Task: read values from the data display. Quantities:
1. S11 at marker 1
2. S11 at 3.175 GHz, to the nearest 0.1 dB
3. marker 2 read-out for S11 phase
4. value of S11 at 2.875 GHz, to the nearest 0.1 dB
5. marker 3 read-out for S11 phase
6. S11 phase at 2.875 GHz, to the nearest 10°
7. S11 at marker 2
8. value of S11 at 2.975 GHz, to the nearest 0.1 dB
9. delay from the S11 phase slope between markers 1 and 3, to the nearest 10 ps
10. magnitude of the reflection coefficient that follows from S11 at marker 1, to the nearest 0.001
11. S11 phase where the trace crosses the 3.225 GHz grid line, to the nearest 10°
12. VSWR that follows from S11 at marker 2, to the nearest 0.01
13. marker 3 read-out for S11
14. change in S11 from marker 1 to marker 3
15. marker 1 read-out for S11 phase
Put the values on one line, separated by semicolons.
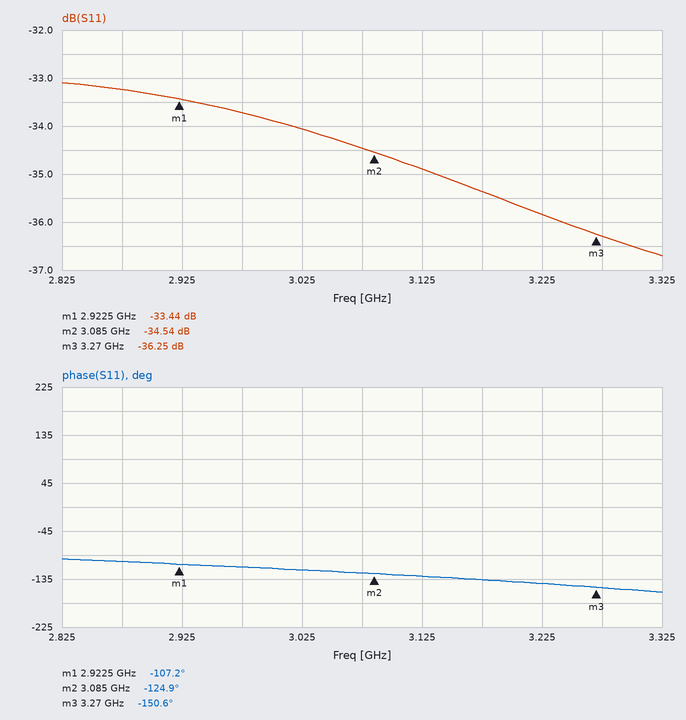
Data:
-33.44 dB; -35.4 dB; -124.9°; -33.2 dB; -150.6°; -100°; -34.54 dB; -33.7 dB; 350 ps; 0.021; -140°; 1.04; -36.25 dB; -2.81 dB; -107.2°
